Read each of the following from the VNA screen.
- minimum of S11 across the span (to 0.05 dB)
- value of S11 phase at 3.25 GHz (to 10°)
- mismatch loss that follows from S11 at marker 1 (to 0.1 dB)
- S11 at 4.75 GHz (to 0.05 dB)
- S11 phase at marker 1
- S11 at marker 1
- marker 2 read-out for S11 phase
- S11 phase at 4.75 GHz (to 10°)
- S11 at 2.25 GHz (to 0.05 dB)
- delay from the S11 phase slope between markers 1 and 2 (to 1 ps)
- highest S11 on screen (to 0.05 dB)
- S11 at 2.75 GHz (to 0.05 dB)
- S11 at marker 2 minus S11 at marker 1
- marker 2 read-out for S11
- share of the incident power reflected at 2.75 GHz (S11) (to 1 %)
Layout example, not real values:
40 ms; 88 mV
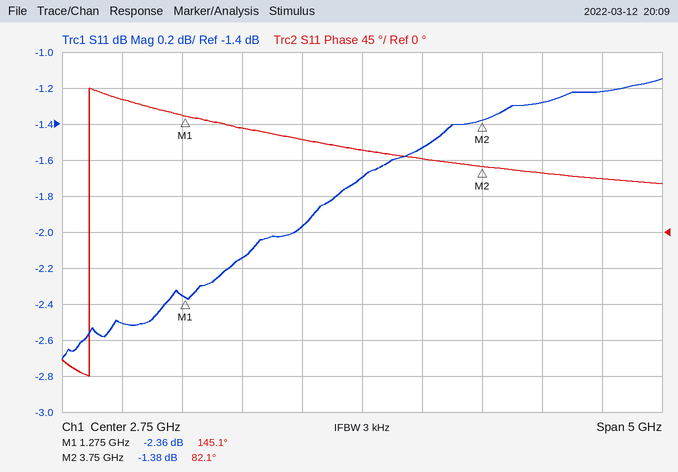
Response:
-2.70 dB; 90°; 3.8 dB; -1.20 dB; 145.1°; -2.36 dB; 82.1°; 70°; -1.95 dB; 71 ps; -1.15 dB; -1.70 dB; 0.98 dB; -1.38 dB; 68 %
